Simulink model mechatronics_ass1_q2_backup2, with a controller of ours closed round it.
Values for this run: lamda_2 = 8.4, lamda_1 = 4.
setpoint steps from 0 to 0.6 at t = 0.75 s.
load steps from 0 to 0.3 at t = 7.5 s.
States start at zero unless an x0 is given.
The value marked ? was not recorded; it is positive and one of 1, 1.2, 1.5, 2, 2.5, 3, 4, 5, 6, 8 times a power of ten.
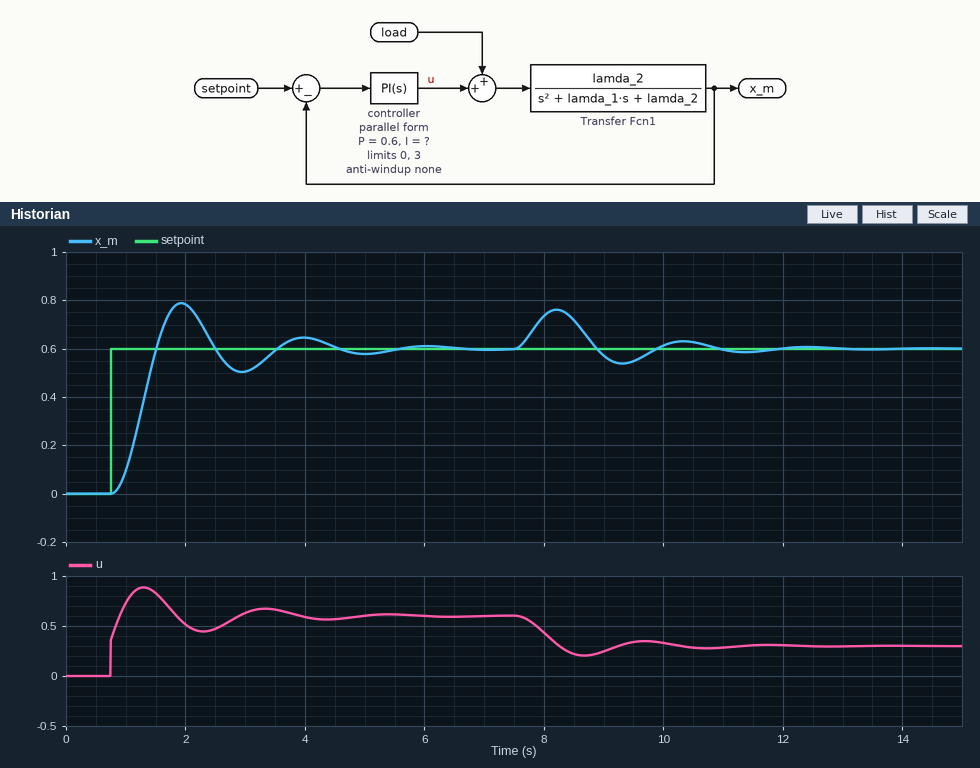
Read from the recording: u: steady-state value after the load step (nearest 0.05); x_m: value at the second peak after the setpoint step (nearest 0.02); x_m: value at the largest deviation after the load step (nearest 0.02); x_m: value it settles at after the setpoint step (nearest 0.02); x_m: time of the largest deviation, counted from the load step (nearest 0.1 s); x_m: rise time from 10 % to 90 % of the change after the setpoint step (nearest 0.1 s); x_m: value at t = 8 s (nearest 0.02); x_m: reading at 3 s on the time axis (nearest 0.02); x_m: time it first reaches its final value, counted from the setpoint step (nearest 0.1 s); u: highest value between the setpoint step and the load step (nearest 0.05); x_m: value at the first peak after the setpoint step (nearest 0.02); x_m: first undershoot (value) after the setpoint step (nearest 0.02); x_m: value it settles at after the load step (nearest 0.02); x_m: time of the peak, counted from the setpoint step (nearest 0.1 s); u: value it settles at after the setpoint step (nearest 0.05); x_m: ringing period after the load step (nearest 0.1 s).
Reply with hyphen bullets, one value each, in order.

- 0.30
- 0.64
- 0.76
- 0.60
- 0.7 s
- 0.5 s
- 0.74
- 0.50
- 0.8 s
- 0.90
- 0.78
- 0.50
- 0.60
- 1.2 s
- 0.60
- 2.1 s
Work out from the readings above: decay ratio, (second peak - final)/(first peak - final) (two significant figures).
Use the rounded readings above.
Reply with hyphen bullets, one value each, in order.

- 0.22
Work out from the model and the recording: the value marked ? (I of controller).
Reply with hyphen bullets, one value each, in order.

- 3
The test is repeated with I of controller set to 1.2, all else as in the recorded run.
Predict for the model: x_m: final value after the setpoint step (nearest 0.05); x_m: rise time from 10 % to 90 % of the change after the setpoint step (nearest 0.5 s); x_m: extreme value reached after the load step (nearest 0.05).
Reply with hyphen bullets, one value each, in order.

- 0.60
- 1.5 s
- 0.80
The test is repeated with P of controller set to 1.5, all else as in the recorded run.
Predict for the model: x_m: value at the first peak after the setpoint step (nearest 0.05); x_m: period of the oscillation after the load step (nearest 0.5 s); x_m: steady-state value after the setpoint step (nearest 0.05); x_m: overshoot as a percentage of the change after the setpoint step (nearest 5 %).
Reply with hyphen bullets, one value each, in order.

- 0.70
- 1.5 s
- 0.60
- 15 %
